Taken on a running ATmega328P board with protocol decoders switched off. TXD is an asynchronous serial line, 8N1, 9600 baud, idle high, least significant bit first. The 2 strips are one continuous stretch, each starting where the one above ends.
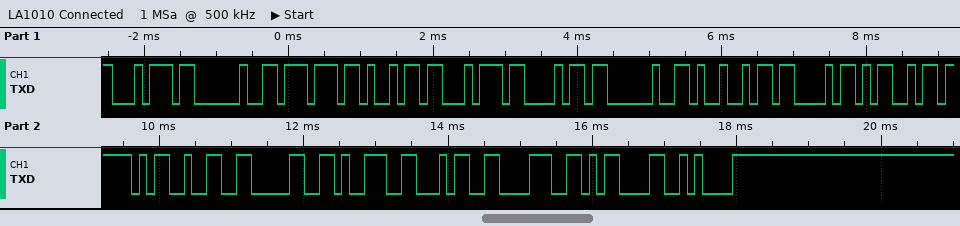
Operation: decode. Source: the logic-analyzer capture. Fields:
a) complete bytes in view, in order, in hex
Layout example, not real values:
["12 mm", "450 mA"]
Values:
["74 20 77 69 74 68 20 49 43 4D 5F 32 30 39 34 38 0D 0A"]
